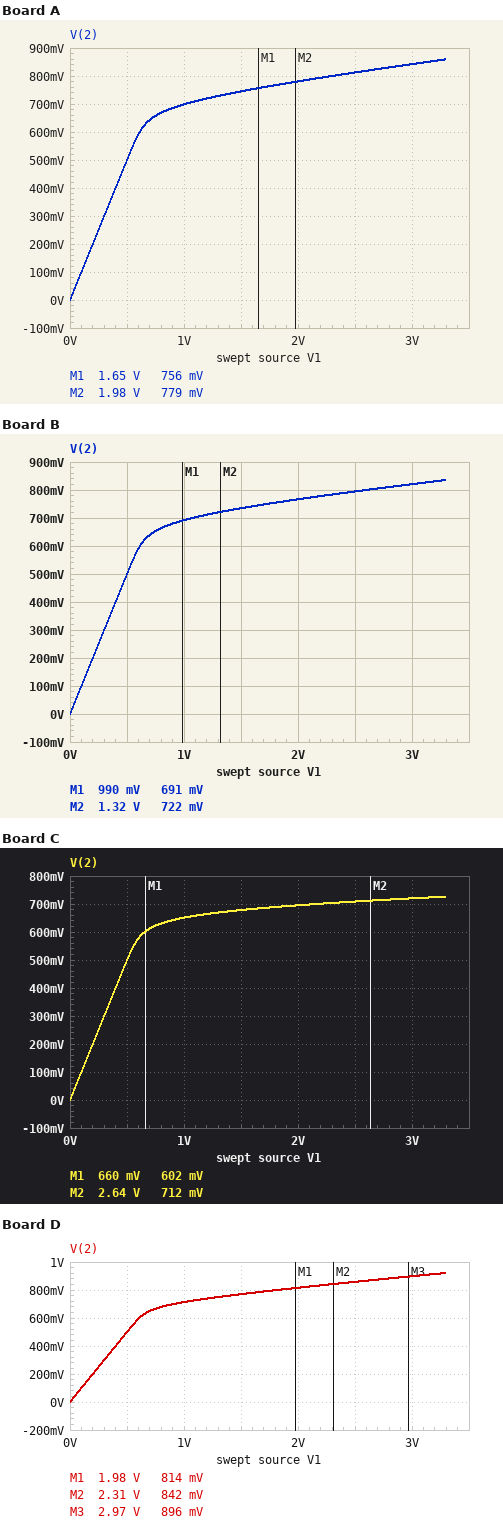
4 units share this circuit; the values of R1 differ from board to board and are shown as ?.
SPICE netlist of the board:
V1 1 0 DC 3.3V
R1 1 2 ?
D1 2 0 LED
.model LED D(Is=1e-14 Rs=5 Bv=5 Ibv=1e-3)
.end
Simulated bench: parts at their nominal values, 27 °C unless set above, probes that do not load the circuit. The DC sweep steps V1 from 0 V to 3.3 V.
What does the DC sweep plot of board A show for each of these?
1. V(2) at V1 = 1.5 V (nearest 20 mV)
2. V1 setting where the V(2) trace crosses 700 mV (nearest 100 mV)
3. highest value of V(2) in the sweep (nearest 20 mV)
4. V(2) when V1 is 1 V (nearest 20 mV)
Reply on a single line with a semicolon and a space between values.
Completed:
740 mV; 1.0 V; 860 mV; 700 mV
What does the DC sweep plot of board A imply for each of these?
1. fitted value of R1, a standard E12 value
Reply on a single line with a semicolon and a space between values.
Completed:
100 Ω
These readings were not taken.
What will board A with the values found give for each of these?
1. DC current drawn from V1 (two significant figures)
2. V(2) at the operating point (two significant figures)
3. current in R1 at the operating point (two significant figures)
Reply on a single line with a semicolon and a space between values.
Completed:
24 mA; 860 mV; 24 mA
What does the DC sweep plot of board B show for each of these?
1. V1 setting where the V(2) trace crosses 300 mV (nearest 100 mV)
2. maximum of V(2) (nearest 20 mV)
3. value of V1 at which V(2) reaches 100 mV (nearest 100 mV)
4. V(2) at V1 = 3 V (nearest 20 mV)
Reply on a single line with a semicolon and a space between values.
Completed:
300 mV; 840 mV; 100 mV; 820 mV
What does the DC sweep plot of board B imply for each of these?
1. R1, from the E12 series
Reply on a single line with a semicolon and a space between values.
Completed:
120 Ω
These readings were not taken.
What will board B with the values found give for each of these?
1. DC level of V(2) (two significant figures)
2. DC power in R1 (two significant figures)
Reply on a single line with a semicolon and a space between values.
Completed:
840 mV; 51 mW
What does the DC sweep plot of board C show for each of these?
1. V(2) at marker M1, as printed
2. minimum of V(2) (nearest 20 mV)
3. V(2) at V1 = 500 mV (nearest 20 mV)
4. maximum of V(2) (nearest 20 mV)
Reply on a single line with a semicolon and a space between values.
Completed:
602 mV; 0 V; 500 mV; 720 mV
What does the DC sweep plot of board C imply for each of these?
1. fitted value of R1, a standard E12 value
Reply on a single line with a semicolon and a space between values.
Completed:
470 Ω
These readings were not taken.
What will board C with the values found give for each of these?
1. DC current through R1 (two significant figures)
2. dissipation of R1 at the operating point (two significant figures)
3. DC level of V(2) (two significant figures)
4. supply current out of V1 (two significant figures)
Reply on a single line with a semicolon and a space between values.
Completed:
5.5 mA; 14 mW; 730 mV; 5.5 mA
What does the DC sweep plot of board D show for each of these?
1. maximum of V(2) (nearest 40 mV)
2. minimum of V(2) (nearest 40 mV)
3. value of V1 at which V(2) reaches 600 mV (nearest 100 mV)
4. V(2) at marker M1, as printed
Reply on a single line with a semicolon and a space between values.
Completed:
920 mV; 0 V; 600 mV; 814 mV
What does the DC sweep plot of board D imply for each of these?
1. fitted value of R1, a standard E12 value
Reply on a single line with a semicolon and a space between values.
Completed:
68 Ω
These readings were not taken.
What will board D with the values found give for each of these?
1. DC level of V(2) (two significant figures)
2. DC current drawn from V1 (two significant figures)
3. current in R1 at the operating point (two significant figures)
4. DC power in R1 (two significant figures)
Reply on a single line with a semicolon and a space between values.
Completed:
920 mV; 35 mA; 35 mA; 83 mW
